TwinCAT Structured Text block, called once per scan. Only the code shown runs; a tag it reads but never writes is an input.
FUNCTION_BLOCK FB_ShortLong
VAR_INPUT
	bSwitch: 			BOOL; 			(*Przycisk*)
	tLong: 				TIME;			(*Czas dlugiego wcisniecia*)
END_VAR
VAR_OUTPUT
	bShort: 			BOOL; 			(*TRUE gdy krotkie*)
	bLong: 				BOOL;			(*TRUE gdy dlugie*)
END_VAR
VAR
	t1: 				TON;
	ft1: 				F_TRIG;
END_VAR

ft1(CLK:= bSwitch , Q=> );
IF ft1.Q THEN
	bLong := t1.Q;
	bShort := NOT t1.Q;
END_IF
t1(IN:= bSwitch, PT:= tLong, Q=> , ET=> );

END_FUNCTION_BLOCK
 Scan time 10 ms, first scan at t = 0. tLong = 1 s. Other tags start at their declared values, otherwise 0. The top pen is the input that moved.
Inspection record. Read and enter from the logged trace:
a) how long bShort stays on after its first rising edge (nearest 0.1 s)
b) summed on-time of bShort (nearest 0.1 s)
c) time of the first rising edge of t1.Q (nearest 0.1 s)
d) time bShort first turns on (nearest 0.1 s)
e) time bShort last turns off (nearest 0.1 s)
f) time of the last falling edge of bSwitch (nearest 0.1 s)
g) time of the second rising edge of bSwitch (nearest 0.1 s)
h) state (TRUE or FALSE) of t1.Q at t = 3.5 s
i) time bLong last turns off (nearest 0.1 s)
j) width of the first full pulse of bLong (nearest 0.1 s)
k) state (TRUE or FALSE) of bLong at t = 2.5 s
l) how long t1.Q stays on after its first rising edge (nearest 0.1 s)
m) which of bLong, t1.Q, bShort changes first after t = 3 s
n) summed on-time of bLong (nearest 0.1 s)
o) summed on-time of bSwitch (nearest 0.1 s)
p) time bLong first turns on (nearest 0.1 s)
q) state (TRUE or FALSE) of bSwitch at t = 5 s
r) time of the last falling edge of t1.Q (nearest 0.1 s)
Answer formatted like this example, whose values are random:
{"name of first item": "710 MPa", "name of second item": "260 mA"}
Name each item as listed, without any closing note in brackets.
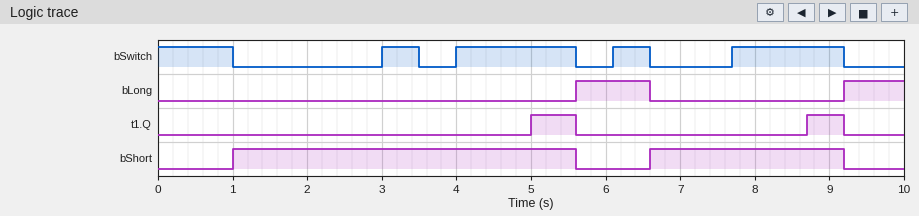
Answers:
{"how long bShort stays on after its first rising edge": "4.6 s", "summed on-time of bShort": "7.2 s", "time of the first rising edge of t1.Q": "5.0 s", "time bShort first turns on": "1.0 s", "time bShort last turns off": "9.2 s", "time of the last falling edge of bSwitch": "9.2 s", "time of the second rising edge of bSwitch": "4.0 s", "state (TRUE or FALSE) of t1.Q at t = 3.5 s": "FALSE", "time bLong last turns off": "6.6 s", "width of the first full pulse of bLong": "1.0 s", "state (TRUE or FALSE) of bLong at t = 2.5 s": "FALSE", "how long t1.Q stays on after its first rising edge": "0.6 s", "which of bLong, t1.Q, bShort changes first after t = 3 s": "t1.Q", "summed on-time of bLong": "1.8 s", "summed on-time of bSwitch": "5.1 s", "time bLong first turns on": "5.6 s", "state (TRUE or FALSE) of bSwitch at t = 5 s": "TRUE", "time of the last falling edge of t1.Q": "9.2 s"}
